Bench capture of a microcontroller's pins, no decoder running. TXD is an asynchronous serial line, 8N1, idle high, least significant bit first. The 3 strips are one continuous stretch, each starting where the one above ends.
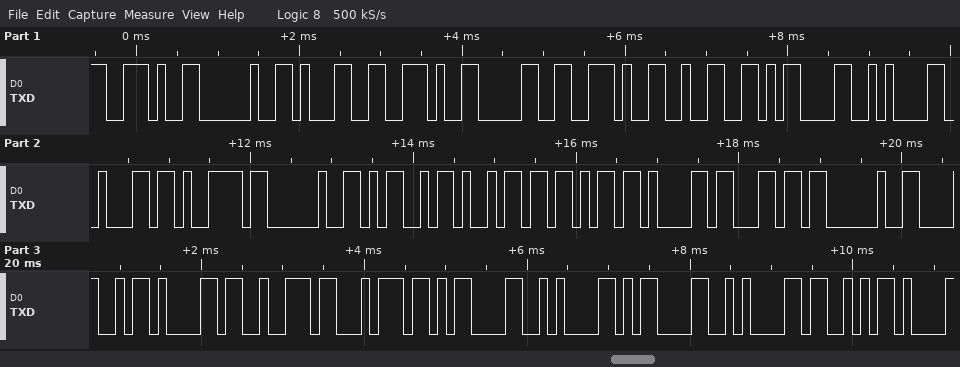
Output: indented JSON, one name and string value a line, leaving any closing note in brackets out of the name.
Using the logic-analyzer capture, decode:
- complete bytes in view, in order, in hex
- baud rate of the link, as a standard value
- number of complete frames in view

{
  "complete bytes in view, in order, in hex": "2E 20 31 2E 30 2E 32 0D 0A 62 79 20 4D 69 6B 61 6C 20 48 61 72 74 0D 0A 0D 0A 53",
  "baud rate of the link, as a standard value": "9600 baud",
  "number of complete frames in view": "27"
}
